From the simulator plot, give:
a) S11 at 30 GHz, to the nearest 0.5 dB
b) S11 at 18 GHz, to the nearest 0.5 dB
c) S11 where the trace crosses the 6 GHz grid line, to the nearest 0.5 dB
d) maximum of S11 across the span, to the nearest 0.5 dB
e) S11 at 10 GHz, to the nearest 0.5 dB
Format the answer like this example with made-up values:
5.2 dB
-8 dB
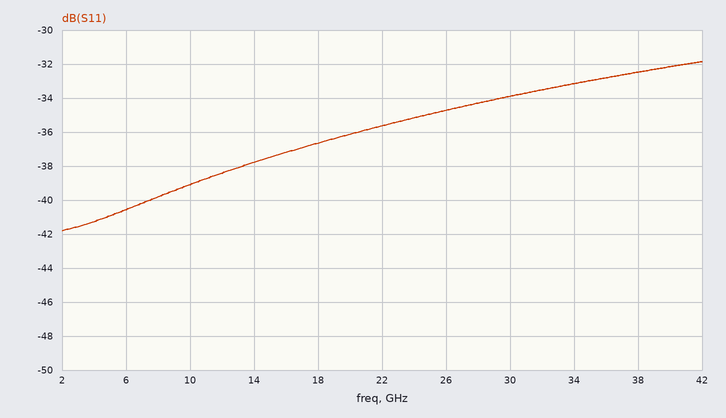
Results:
-34.0 dB
-36.5 dB
-40.5 dB
-32.0 dB
-39.0 dB
